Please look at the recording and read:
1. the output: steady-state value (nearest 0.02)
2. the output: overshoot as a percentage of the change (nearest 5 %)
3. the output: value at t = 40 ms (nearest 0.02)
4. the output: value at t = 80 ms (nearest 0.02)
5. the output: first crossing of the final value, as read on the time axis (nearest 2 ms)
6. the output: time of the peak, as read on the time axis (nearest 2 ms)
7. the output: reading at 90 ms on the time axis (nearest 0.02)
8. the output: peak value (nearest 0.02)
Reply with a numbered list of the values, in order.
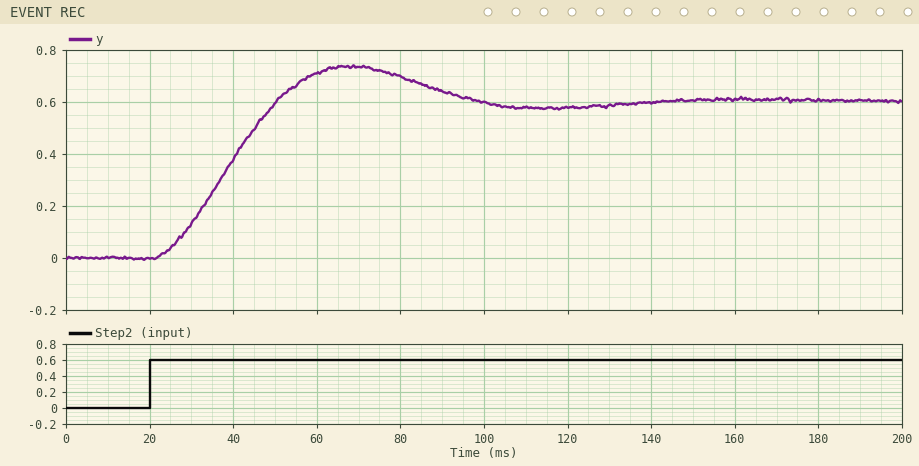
1. 0.60
2. 20 %
3. 0.38
4. 0.70
5. 50 ms
6. 68 ms
7. 0.64
8. 0.74
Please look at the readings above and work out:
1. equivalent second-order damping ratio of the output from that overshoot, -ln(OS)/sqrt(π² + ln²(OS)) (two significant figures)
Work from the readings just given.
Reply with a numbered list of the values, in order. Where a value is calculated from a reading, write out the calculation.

1. ln(0.2) = -1.609; 1.609 / sqrt(9.870 + 2.590) = 0.46
